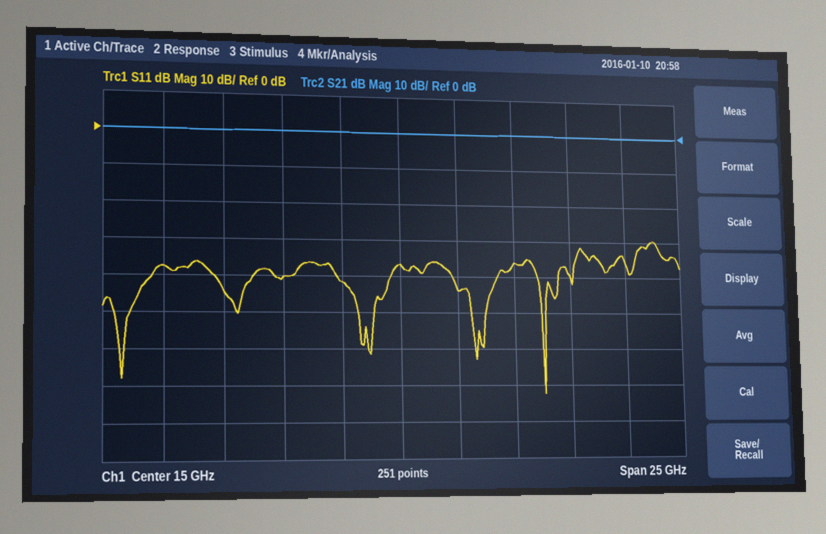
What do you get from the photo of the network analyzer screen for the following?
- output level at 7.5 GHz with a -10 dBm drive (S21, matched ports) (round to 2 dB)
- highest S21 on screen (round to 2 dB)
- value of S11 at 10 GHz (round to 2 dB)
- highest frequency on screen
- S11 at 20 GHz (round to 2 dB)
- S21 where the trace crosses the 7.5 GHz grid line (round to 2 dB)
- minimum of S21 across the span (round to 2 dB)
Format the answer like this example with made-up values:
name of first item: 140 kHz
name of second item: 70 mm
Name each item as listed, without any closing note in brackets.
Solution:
output level at 7.5 GHz with a -10 dBm drive (S21, matched ports): -10 dBm
highest S21 on screen: 0 dB
value of S11 at 10 GHz: -40 dB
highest frequency on screen: 27.5 GHz
S11 at 20 GHz: -36 dB
S21 where the trace crosses the 7.5 GHz grid line: 0 dB
minimum of S21 across the span: 0 dB
